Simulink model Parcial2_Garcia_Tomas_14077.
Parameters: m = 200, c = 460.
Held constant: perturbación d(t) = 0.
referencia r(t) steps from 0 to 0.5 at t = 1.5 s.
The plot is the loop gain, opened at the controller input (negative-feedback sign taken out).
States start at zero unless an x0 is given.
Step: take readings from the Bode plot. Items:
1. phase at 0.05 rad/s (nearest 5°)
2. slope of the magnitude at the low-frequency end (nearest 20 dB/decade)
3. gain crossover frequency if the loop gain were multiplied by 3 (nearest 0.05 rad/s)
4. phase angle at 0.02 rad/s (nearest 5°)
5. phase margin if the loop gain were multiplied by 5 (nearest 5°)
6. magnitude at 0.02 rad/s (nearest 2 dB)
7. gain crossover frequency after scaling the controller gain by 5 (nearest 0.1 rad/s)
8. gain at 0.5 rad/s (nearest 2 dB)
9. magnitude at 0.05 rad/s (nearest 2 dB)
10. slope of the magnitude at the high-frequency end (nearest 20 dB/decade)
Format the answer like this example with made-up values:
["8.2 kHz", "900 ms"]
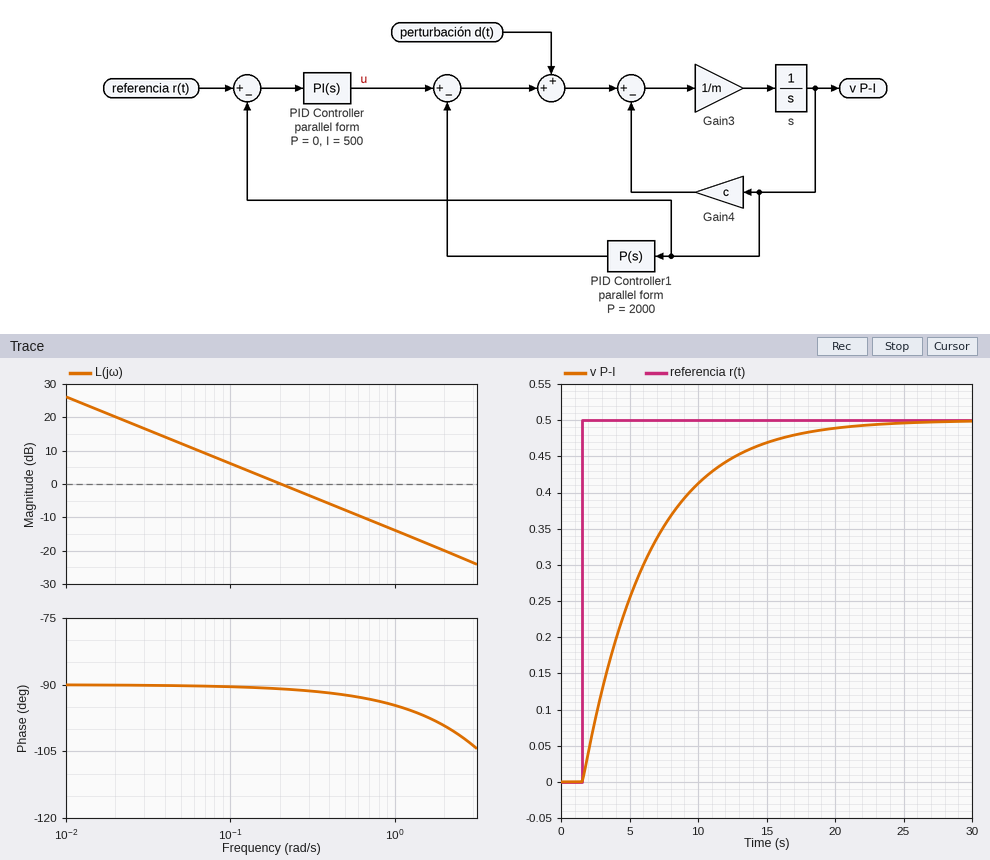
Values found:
["-90°", "-20 dB/decade", "0.60 rad/s", "-90°", "85°", "20 dB", "1.0 rad/s", "-8 dB", "12 dB", "-20 dB/decade"]
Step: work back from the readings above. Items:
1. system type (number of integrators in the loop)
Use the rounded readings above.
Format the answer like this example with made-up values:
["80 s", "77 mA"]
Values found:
["1"]
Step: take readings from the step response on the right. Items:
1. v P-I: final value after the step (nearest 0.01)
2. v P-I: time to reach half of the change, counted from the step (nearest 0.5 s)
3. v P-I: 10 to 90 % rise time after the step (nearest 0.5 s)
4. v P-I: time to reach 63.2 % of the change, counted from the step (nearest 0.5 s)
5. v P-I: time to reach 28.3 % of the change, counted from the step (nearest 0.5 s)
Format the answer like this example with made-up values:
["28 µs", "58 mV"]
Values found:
["0.50", "3.5 s", "10.5 s", "5.0 s", "1.5 s"]
